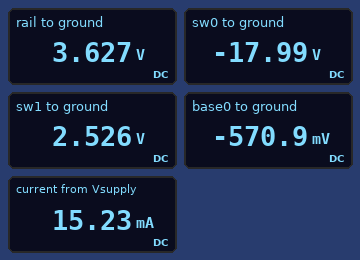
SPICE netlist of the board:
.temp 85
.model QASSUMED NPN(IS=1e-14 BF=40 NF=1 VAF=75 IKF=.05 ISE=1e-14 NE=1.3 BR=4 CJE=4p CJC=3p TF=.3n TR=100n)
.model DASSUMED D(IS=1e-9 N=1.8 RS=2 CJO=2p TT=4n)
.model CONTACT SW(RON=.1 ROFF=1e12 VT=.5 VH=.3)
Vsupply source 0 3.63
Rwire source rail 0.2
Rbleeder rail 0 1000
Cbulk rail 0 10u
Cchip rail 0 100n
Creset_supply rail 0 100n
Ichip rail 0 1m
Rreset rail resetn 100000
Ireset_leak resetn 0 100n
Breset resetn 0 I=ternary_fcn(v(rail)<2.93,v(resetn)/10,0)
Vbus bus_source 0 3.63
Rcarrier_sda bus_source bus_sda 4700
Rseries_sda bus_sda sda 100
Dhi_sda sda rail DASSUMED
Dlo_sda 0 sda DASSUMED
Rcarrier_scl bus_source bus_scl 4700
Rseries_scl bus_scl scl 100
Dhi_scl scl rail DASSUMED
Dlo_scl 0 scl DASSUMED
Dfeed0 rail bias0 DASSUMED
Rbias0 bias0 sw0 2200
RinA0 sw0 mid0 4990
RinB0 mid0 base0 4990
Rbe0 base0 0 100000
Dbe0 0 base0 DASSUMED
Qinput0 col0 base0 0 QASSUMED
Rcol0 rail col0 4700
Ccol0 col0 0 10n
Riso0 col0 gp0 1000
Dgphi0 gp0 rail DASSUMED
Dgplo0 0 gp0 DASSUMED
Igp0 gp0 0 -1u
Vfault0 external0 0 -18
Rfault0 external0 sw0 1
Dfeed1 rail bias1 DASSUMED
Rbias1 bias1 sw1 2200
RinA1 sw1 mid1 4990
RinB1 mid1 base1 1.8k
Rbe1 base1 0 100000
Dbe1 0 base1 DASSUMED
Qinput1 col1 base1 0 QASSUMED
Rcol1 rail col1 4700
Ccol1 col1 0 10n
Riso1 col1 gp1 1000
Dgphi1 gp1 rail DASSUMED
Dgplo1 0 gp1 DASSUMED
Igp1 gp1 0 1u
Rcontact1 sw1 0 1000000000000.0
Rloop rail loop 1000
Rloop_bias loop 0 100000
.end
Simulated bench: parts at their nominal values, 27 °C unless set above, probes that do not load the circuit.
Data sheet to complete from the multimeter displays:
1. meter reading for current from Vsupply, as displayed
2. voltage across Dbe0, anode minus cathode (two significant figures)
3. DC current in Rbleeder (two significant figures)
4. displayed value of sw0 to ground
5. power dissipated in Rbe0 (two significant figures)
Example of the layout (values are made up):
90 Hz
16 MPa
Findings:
15.23 mA
570 mV
3.6 mA
-17.99 V
3.3 µW
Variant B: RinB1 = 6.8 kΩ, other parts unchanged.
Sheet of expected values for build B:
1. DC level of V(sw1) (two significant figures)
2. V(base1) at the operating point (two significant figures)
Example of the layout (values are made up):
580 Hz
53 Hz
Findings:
2.8 V
560 mV
